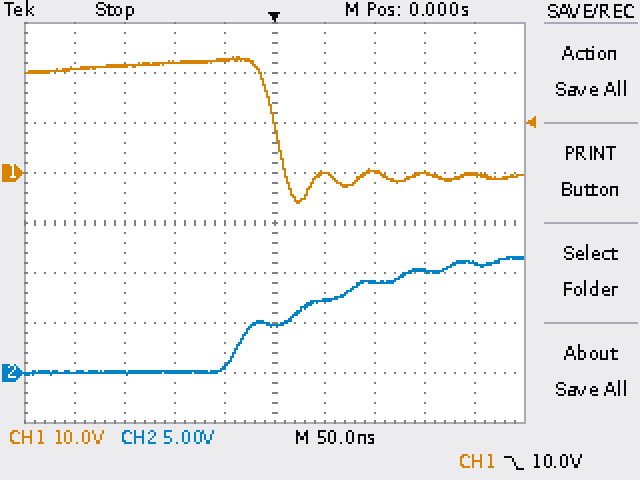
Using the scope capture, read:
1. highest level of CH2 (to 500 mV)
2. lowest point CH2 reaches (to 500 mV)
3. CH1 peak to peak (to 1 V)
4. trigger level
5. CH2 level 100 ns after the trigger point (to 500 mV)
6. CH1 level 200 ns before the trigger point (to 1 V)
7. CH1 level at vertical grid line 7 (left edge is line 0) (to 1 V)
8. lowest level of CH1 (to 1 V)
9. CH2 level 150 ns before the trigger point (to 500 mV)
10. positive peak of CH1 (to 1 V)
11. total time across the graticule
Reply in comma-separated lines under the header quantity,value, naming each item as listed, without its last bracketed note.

quantity,value
highest level of CH2,11.5 V
lowest point CH2 reaches,0.0 V
CH1 peak to peak,29 V
trigger level,10.0 V
CH2 level 100 ns after the trigger point,9.0 V
CH1 level 200 ns before the trigger point,21 V
CH1 level at vertical grid line 7 (left edge is line 0),0 V
lowest level of CH1,-6 V
CH2 level 150 ns before the trigger point,0.0 V
positive peak of CH1,23 V
total time across the graticule,500 ns
